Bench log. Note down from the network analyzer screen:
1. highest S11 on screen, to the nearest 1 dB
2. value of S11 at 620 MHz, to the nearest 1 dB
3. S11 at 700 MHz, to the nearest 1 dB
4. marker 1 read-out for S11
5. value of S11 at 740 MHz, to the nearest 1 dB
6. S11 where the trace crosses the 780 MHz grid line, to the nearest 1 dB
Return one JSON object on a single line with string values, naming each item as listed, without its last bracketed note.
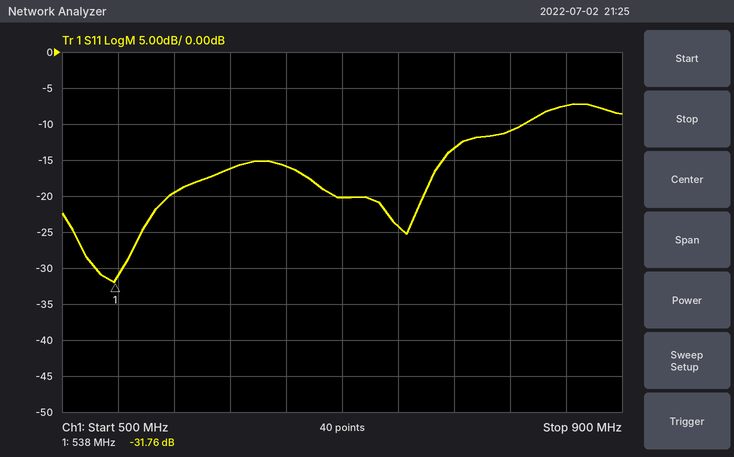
{"highest S11 on screen, to the nearest 1 dB": "-7 dB", "value of S11 at 620 MHz, to the nearest 1 dB": "-16 dB", "S11 at 700 MHz, to the nearest 1 dB": "-20 dB", "marker 1 read-out for S11": "-31.76 dB", "value of S11 at 740 MHz, to the nearest 1 dB": "-24 dB", "S11 where the trace crosses the 780 MHz grid line, to the nearest 1 dB": "-13 dB"}
